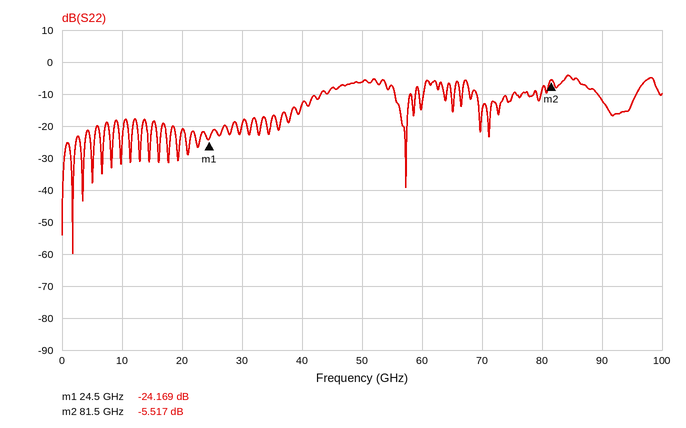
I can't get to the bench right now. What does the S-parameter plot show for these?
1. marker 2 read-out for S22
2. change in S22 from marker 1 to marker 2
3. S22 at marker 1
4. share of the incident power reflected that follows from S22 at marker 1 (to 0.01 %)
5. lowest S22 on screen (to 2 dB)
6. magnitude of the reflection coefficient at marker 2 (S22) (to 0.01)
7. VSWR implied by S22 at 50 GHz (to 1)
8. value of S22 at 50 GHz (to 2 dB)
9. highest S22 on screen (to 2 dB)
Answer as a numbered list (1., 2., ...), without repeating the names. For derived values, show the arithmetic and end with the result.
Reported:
1. -5.517 dB
2. -5.517 − (-24.169) = 18.652 dB
3. -24.169 dB
4. 10^(-24.169/10) ≈ 0.38 %
5. -60 dB
6. 10^(-5.517/20) ≈ 0.53
7. |Γ| = 10^(-6/20) = 0.5012; VSWR = (1 + 0.5012)/(1 − 0.5012) ≈ 3
8. -6 dB
9. -4 dB
